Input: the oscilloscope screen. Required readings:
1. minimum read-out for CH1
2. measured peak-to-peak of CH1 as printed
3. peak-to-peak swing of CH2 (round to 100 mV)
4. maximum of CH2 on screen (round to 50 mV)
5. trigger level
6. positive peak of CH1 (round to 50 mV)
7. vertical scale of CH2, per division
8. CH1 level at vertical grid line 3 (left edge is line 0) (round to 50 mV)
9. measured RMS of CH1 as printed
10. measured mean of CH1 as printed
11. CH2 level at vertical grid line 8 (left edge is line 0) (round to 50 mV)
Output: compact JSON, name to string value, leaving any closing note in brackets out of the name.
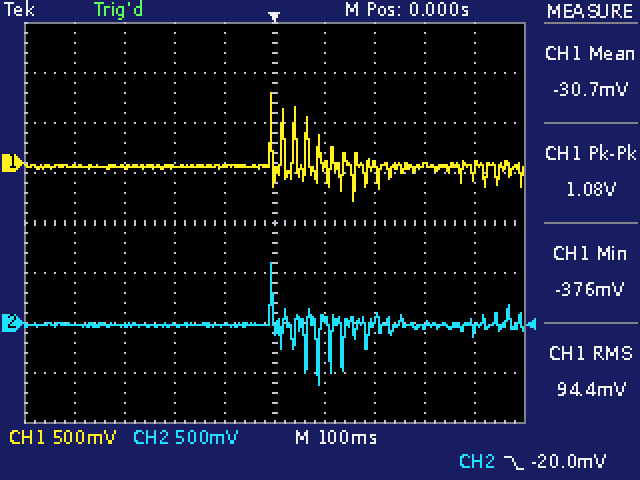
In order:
{"minimum read-out for CH1": "-376 mV", "measured peak-to-peak of CH1 as printed": "1.08 V", "peak-to-peak swing of CH2": "1.20 V", "maximum of CH2 on screen": "600 mV", "trigger level": "-20.0 mV", "positive peak of CH1": "700 mV", "vertical scale of CH2, per division": "500 mV", "CH1 level at vertical grid line 3 (left edge is line 0)": "-50 mV", "measured RMS of CH1 as printed": "94.4 mV", "measured mean of CH1 as printed": "-30.7 mV", "CH2 level at vertical grid line 8 (left edge is line 0)": "0 mV"}
